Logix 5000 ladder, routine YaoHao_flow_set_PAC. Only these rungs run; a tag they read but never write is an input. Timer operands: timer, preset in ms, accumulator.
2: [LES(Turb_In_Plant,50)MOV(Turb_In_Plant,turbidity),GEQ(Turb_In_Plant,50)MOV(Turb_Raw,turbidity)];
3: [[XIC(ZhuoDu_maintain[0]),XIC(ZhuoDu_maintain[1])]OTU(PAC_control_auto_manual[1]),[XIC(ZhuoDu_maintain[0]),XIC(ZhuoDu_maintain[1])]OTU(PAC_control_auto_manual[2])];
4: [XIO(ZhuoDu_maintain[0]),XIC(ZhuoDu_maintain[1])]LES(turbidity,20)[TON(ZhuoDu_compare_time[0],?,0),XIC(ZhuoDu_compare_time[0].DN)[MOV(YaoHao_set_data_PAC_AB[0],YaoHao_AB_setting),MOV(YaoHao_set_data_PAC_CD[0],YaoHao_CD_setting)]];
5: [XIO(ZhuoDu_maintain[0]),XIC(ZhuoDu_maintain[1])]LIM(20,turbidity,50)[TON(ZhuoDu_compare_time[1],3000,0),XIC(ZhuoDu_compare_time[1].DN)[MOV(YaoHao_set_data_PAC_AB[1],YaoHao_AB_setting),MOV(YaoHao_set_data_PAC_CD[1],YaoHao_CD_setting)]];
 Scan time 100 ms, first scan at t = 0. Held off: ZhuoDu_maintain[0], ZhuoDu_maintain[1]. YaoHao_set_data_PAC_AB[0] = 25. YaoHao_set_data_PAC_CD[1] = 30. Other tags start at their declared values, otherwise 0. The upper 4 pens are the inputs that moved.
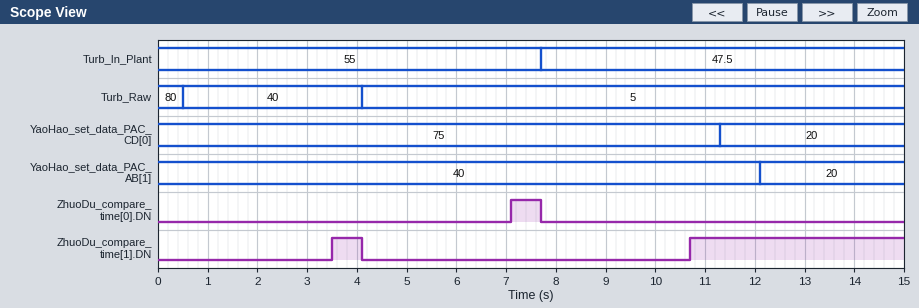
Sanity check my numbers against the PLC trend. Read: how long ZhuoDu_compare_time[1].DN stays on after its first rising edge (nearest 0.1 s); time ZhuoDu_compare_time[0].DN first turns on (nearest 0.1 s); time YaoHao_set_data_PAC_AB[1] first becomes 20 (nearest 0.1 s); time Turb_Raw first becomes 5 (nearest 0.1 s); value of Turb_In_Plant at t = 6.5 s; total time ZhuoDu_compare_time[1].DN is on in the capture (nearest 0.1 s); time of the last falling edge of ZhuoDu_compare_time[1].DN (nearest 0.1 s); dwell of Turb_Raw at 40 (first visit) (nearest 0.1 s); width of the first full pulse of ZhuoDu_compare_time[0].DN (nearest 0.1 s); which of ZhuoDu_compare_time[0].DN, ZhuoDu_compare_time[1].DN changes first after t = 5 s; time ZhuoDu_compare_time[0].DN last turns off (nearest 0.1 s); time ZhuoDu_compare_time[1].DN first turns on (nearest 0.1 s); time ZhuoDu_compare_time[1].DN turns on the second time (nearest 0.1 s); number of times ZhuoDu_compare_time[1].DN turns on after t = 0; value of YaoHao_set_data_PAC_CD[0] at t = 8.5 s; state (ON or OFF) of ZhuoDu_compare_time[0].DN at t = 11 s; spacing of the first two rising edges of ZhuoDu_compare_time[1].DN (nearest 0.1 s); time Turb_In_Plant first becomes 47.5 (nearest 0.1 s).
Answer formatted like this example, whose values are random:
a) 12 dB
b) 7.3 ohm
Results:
a) 0.6 s
b) 7.1 s
c) 12.1 s
d) 4.1 s
e) 55
f) 4.9 s
g) 4.1 s
h) 3.6 s
i) 0.6 s
j) ZhuoDu_compare_time[0].DN
k) 7.7 s
l) 3.5 s
m) 10.7 s
n) 2
o) 75
p) OFF
q) 7.2 s
r) 7.7 s
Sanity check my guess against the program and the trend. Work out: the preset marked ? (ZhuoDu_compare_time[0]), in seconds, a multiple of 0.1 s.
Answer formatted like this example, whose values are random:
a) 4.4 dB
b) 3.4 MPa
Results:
a) 3.0 s
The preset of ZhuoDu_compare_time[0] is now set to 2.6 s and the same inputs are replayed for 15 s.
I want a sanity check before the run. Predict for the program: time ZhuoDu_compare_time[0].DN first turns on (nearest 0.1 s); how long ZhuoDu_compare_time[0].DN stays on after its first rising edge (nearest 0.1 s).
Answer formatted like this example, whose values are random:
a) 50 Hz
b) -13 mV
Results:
a) 6.7 s
b) 1.0 s
